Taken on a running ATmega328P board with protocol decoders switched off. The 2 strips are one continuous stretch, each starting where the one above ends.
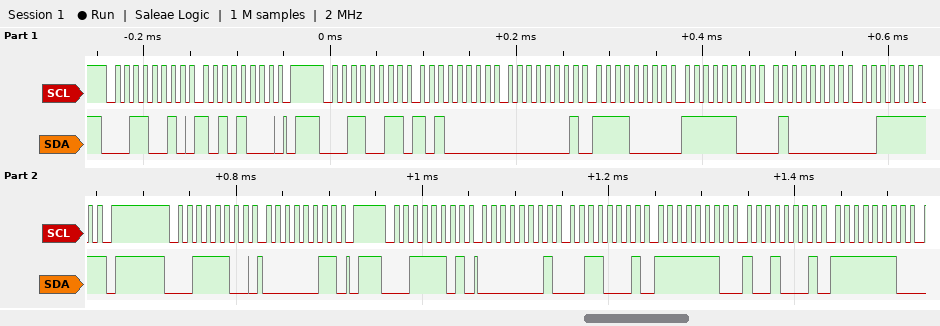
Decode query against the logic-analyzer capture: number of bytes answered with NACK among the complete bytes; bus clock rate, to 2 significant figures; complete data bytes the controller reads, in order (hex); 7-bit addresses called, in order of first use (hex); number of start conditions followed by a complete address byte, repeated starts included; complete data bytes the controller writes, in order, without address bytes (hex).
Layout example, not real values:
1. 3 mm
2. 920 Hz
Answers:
1. 1
2. 100 kHz
3. A0 01 F0 FC 40 3F 01 31 FE 91 FE
4. 0x19 0x1E
5. 4
6. A8 03
